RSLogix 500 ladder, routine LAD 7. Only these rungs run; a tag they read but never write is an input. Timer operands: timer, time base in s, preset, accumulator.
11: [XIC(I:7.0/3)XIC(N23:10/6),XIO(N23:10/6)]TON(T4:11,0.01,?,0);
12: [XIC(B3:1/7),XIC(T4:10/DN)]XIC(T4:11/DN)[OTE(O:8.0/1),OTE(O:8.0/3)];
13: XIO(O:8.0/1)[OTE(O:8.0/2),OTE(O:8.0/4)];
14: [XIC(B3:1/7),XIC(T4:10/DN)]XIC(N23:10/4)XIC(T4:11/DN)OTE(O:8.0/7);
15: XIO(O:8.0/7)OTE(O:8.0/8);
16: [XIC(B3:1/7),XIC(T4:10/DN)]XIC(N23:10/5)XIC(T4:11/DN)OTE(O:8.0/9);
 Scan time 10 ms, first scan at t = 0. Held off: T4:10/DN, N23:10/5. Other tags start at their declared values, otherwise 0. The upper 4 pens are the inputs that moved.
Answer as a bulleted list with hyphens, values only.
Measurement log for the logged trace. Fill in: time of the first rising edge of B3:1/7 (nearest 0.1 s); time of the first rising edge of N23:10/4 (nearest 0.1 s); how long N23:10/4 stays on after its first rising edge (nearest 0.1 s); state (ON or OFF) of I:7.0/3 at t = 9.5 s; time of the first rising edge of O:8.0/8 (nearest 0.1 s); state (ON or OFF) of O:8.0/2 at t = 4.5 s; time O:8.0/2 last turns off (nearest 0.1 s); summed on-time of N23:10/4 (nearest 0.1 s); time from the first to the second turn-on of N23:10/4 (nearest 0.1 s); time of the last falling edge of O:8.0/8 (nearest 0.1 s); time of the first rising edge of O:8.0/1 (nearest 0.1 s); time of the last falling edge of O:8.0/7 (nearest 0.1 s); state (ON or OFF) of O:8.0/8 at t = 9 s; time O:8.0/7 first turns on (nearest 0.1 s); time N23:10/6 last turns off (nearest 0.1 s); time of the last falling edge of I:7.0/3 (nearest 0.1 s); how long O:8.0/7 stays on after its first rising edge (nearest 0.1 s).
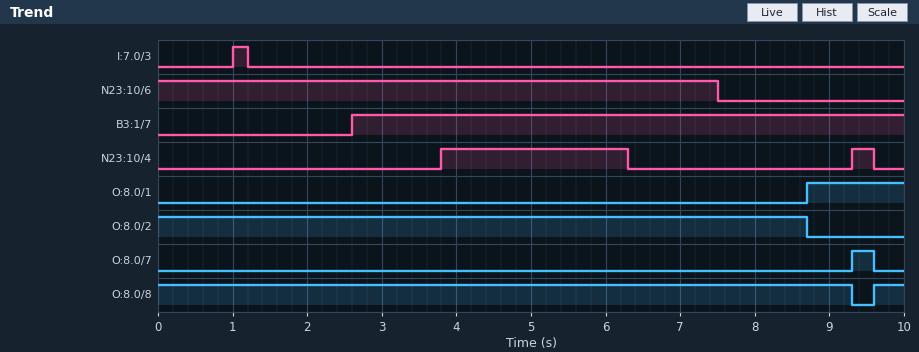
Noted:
- 2.6 s
- 3.8 s
- 2.5 s
- OFF
- 9.6 s
- ON
- 8.7 s
- 2.8 s
- 5.5 s
- 9.3 s
- 8.7 s
- 9.6 s
- ON
- 9.3 s
- 7.5 s
- 1.2 s
- 0.3 s
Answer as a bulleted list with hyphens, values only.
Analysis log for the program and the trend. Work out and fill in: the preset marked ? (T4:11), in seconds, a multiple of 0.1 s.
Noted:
- 1.2 s
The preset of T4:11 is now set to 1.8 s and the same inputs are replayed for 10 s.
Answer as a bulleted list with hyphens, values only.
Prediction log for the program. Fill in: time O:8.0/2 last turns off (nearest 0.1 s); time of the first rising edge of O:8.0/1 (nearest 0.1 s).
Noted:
- 9.3 s
- 9.3 s
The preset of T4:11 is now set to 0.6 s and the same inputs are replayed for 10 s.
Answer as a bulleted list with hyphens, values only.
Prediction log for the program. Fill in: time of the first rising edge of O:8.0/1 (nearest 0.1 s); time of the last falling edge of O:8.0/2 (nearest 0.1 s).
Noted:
- 8.1 s
- 8.1 s
